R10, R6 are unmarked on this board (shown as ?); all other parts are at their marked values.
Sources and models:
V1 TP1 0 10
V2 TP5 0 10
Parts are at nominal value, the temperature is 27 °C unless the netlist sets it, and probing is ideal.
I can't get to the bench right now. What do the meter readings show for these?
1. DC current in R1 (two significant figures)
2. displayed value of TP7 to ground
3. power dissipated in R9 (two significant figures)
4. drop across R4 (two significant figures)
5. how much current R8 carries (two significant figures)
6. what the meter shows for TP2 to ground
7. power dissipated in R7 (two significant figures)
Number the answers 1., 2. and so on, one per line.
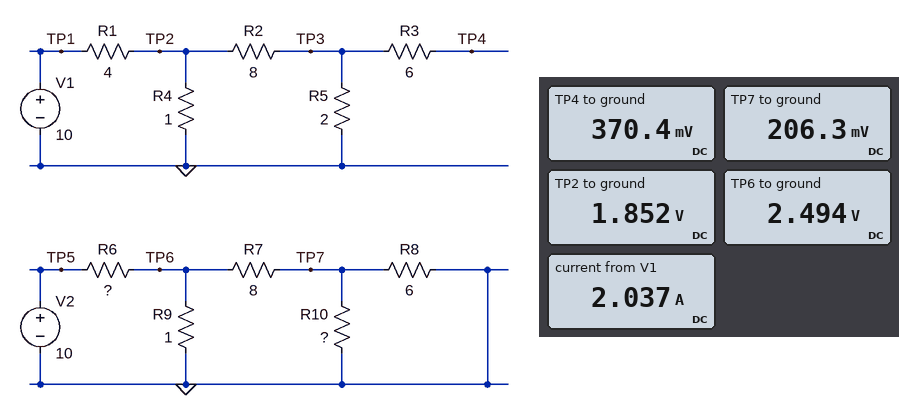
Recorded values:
1. 2.0 A
2. 206.3 mV
3. 6.2 W
4. 1.9 V
5. 34 mA
6. 1.852 V
7. 650 mW
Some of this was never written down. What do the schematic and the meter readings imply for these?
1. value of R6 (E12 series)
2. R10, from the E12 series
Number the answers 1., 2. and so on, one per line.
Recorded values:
1. 2.7 Ω
2. 0.82 Ω
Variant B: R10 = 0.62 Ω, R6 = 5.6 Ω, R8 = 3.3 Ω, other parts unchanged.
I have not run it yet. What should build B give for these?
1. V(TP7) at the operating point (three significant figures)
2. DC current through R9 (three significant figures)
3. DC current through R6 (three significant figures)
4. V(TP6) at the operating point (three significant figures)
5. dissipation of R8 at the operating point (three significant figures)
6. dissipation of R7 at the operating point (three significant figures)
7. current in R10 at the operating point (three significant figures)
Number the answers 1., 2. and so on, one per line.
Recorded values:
1. 84.4 mV
2. 1.38 A
3. 1.54 A
4. 1.38 V
5. 2.16 mW
6. 209 mW
7. 136 mA
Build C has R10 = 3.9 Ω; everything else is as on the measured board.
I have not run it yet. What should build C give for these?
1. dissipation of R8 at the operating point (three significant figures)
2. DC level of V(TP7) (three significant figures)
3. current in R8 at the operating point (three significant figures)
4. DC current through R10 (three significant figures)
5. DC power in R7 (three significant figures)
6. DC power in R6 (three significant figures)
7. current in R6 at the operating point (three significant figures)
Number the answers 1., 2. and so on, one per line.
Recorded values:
1. 55.3 mW
2. 576 mV
3. 96.0 mA
4. 148 mA
5. 475 mW
6. 20.7 W
7. 2.77 A
